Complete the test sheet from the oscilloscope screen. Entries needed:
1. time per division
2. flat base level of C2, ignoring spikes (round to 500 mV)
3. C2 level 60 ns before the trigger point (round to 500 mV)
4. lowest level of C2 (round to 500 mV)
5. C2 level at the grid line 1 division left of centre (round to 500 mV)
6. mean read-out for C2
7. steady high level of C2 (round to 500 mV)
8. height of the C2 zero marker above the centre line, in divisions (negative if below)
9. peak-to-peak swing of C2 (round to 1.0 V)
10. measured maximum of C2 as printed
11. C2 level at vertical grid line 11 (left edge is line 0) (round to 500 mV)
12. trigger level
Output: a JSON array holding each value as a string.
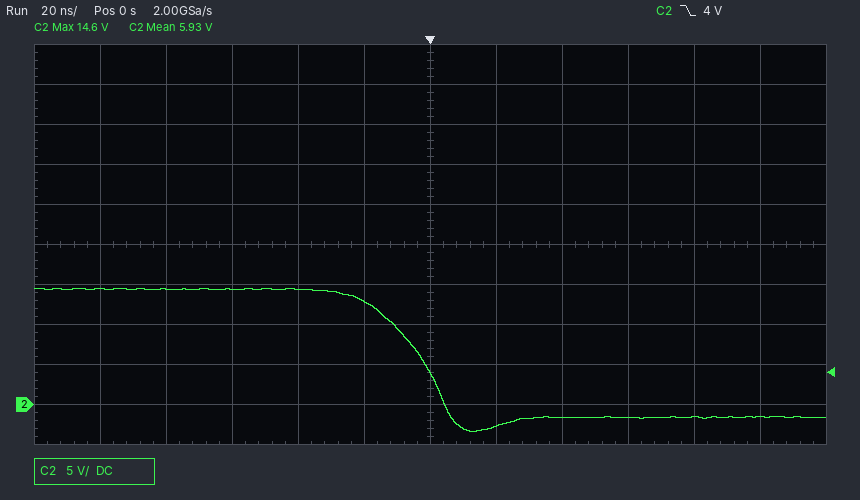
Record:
["20 ns", "-1.5 V", "14.5 V", "-3.5 V", "13.0 V", "5.93 V", "14.5 V", "-4.0 div", "18.0 V", "14.6 V", "-1.5 V", "4 V"]
